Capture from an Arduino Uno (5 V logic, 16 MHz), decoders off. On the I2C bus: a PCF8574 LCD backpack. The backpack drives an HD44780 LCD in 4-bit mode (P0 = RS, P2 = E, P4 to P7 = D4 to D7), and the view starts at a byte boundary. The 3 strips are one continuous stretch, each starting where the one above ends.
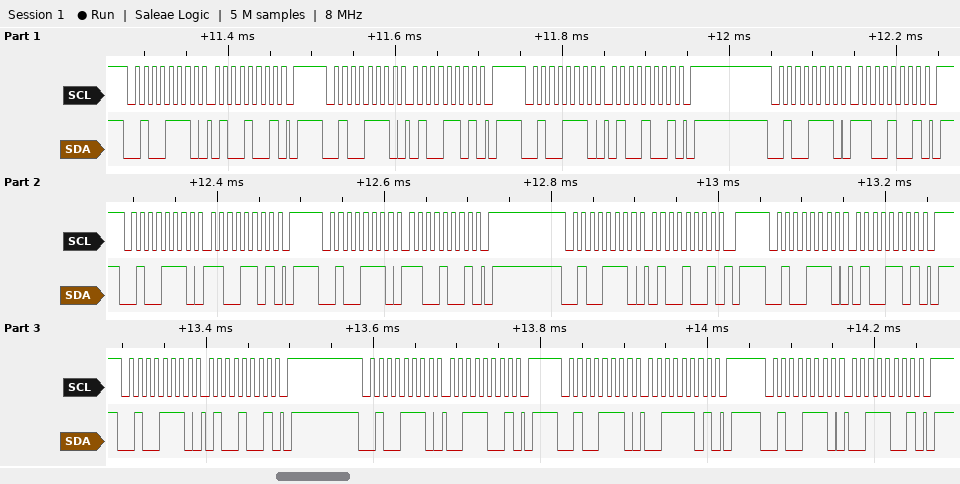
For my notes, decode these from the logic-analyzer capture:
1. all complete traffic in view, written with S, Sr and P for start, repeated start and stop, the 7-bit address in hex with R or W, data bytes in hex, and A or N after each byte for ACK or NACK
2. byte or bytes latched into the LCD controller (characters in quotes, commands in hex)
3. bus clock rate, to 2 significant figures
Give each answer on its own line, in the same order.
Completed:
S 27W A 49 A P S 27W A 4D A P S 27W A 49 A P S 27W A C9 A P S 27W A CD A P S 27W A C9 A P S 27W A 49 A P S 27W A 4D A P S 27W A 49 A P S 27W A 39 A P S 27W A 3D A P S 27W A 39 A P
'L' 'C'
100 kHz
